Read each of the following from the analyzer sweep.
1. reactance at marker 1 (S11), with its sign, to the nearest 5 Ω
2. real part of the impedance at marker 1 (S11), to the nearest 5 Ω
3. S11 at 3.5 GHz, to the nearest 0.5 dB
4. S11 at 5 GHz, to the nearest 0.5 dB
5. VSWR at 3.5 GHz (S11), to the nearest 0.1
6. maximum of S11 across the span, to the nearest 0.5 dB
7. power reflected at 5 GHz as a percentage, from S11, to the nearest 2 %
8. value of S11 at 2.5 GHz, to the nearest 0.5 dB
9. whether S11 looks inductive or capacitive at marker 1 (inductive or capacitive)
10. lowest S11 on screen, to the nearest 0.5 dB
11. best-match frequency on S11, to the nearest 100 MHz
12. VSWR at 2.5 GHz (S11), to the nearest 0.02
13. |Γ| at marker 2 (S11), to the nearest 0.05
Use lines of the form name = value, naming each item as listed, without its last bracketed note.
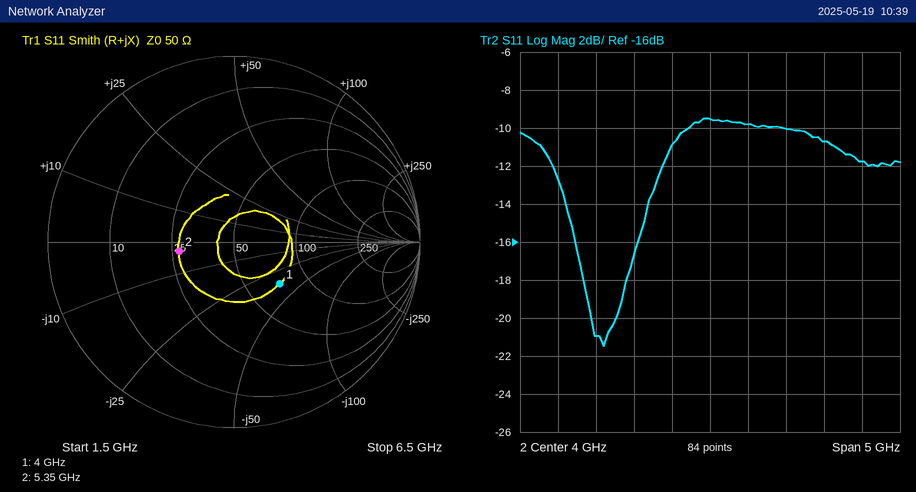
reactance at marker 1 (S11), with its sign, to the nearest 5 Ω = -35 Ω
real part of the impedance at marker 1 (S11), to the nearest 5 Ω = 70 Ω
S11 at 3.5 GHz, to the nearest 0.5 dB = -11.0 dB
S11 at 5 GHz, to the nearest 0.5 dB = -10.0 dB
VSWR at 3.5 GHz (S11), to the nearest 0.1 = 1.8
maximum of S11 across the span, to the nearest 0.5 dB = -9.5 dB
power reflected at 5 GHz as a percentage, from S11, to the nearest 2 % = 10 %
value of S11 at 2.5 GHz, to the nearest 0.5 dB = -21.0 dB
whether S11 looks inductive or capacitive at marker 1 = capacitive
lowest S11 on screen, to the nearest 0.5 dB = -21.5 dB
best-match frequency on S11, to the nearest 100 MHz = 2.6 GHz
VSWR at 2.5 GHz (S11), to the nearest 0.02 = 1.20
|Γ| at marker 2 (S11), to the nearest 0.05 = 0.30
